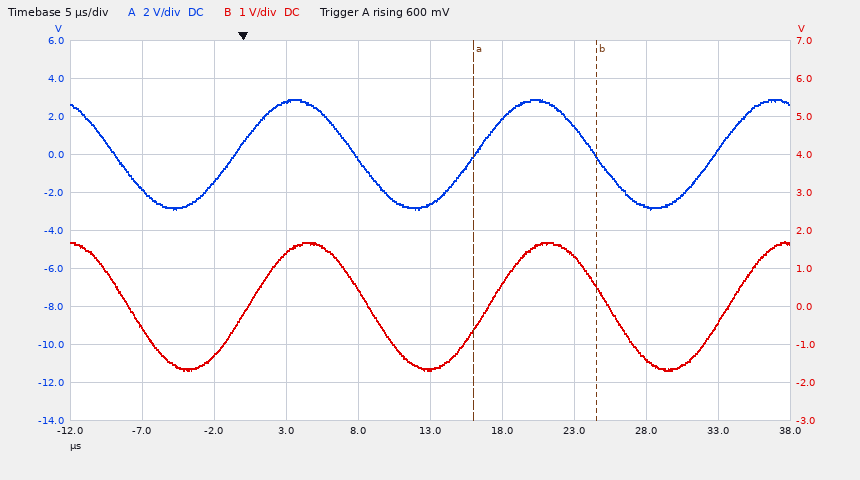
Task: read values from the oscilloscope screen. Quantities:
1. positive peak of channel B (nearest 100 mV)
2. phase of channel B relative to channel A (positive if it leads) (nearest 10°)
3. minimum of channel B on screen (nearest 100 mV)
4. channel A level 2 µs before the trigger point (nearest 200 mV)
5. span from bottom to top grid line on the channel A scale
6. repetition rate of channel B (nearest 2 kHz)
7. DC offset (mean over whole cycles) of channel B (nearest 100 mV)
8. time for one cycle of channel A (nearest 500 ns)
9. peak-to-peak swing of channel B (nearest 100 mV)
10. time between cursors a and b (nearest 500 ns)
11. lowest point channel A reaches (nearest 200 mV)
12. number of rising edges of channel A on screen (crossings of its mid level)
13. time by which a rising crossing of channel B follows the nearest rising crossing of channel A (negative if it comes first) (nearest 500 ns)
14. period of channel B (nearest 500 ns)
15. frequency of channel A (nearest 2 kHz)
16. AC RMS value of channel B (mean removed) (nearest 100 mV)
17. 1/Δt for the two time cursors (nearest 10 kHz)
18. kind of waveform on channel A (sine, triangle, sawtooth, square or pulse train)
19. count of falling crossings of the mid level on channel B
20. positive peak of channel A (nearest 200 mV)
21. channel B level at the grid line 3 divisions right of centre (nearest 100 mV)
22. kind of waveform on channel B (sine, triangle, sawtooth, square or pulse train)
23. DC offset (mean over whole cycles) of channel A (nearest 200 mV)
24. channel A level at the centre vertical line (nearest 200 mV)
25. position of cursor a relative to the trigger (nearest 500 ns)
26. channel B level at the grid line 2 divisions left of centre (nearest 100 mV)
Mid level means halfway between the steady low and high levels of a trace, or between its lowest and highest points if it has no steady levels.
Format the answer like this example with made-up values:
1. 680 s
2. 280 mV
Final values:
1. 1.7 V
2. -20°
3. -1.7 V
4. -1.4 V
5. 20 V
6. 60 kHz
7. 0.0 V
8. 16.5 µs
9. 3.4 V
10. 8.5 µs
11. -2.8 V
12. 3
13. +1.0 µs
14. 16.5 µs
15. 60 kHz
16. 1.2 V
17. 120 kHz
18. sine
19. 3
20. 2.8 V
21. -1.4 V
22. sine
23. 0.0 V
24. -2.6 V
25. +16.0 µs
26. 1.4 V
